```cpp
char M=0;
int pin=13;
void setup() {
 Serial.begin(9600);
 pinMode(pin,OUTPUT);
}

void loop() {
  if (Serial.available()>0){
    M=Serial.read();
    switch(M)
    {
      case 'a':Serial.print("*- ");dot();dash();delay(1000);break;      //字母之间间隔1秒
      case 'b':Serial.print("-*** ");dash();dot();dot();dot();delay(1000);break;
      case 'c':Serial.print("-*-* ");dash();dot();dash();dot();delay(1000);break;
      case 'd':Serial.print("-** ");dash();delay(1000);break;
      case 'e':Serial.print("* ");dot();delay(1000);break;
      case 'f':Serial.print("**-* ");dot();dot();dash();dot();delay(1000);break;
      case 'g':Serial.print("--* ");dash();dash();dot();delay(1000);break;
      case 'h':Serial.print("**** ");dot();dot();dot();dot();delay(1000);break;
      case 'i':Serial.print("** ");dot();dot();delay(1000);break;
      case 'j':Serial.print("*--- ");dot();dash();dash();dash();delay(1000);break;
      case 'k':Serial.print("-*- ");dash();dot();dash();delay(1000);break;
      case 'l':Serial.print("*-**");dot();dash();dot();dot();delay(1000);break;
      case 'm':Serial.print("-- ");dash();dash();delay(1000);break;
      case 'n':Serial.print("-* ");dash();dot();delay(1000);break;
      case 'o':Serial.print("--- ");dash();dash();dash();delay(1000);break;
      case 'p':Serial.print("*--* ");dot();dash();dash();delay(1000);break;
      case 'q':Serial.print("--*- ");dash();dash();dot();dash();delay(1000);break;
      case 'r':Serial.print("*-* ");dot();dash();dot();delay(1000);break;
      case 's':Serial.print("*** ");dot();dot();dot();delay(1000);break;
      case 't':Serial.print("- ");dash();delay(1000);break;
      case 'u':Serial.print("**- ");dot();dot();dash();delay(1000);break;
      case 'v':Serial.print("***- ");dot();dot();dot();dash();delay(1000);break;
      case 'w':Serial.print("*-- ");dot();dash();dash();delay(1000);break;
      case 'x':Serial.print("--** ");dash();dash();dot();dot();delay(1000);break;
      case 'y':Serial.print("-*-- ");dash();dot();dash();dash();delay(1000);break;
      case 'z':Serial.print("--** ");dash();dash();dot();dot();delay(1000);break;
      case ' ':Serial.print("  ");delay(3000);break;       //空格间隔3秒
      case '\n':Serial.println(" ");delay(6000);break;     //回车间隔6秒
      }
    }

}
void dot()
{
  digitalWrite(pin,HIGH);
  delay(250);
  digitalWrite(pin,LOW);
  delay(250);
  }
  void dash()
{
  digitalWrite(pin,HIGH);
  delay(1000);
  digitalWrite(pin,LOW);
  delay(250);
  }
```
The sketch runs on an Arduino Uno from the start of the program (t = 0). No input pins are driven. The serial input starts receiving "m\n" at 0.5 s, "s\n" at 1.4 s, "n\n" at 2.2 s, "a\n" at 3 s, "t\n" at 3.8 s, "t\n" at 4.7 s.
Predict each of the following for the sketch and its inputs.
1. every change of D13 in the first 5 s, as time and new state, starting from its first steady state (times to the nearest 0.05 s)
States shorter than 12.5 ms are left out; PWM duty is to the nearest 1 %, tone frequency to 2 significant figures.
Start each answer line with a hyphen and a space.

- 0 s low; 0.5 s high; 1.5 s low; 1.75 s high; 2.75 s low
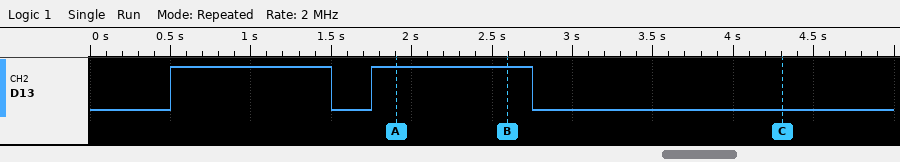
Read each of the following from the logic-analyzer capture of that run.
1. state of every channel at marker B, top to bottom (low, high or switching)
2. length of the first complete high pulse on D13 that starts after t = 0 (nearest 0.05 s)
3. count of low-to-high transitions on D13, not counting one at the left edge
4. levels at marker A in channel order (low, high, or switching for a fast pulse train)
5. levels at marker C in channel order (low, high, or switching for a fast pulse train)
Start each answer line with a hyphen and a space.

- D13 high
- 1.00 s
- 2
- D13 high
- D13 low
